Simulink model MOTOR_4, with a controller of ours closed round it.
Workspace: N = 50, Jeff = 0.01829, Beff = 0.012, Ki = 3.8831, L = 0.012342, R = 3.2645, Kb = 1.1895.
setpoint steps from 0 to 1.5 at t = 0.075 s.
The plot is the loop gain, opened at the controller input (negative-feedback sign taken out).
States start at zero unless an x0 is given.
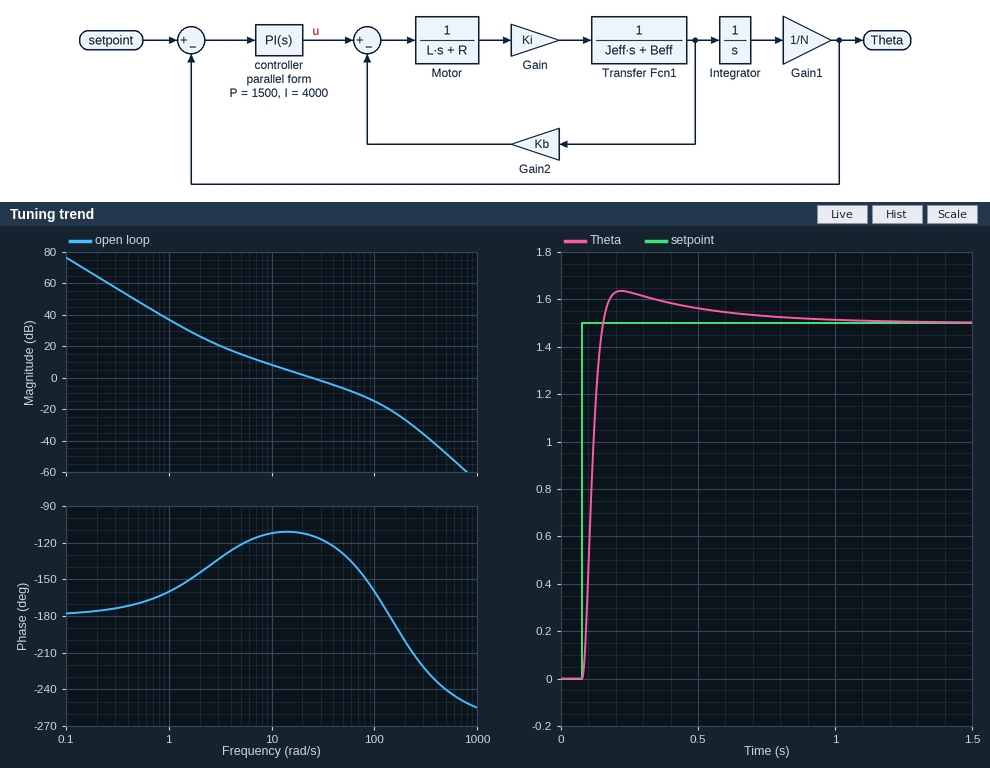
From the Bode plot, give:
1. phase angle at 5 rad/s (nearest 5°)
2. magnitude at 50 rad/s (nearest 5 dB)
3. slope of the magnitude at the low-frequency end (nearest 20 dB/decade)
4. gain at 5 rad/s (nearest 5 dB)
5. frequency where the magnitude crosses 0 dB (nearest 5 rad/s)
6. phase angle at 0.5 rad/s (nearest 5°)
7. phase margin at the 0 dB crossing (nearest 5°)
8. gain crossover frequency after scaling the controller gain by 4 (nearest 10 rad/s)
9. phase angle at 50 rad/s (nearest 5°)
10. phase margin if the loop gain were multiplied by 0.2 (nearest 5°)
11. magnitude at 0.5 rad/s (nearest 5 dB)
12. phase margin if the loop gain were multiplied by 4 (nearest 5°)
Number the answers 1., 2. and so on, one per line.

1. -120°
2. -5 dB
3. -40 dB/decade
4. 15 dB
5. 25 rad/s
6. -170°
7. 65°
8. 80 rad/s
9. -130°
10. 60°
11. 50 dB
12. 30°
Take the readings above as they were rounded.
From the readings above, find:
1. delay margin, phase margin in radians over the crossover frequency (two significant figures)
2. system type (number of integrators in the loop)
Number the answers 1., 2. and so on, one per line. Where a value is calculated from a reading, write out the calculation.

1. 65 × π / 180 / 25 = 0.045 s
2. 2
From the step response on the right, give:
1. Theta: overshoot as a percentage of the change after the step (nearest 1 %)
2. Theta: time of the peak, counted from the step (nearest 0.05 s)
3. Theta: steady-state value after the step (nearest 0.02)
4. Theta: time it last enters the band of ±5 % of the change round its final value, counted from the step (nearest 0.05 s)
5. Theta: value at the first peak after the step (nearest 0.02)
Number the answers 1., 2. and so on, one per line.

1. 9 %
2. 0.15 s
3. 1.50
4. 0.35 s
5. 1.64
